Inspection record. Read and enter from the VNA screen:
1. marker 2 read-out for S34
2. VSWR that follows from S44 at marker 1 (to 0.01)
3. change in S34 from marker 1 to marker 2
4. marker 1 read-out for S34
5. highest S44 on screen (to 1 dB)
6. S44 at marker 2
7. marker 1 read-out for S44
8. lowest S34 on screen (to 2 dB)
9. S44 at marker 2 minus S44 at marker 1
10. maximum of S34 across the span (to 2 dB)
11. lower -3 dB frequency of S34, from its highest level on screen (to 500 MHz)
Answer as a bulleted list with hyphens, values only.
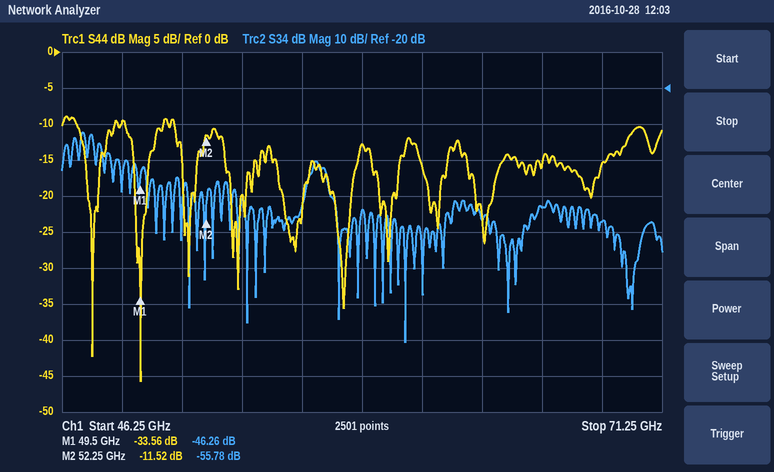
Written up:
- -55.78 dB
- 1.04
- -9.52 dB
- -46.26 dB
- -9 dB
- -11.52 dB
- -33.56 dB
- -90 dB
- 22.04 dB
- -32 dB
- 47.0 GHz
